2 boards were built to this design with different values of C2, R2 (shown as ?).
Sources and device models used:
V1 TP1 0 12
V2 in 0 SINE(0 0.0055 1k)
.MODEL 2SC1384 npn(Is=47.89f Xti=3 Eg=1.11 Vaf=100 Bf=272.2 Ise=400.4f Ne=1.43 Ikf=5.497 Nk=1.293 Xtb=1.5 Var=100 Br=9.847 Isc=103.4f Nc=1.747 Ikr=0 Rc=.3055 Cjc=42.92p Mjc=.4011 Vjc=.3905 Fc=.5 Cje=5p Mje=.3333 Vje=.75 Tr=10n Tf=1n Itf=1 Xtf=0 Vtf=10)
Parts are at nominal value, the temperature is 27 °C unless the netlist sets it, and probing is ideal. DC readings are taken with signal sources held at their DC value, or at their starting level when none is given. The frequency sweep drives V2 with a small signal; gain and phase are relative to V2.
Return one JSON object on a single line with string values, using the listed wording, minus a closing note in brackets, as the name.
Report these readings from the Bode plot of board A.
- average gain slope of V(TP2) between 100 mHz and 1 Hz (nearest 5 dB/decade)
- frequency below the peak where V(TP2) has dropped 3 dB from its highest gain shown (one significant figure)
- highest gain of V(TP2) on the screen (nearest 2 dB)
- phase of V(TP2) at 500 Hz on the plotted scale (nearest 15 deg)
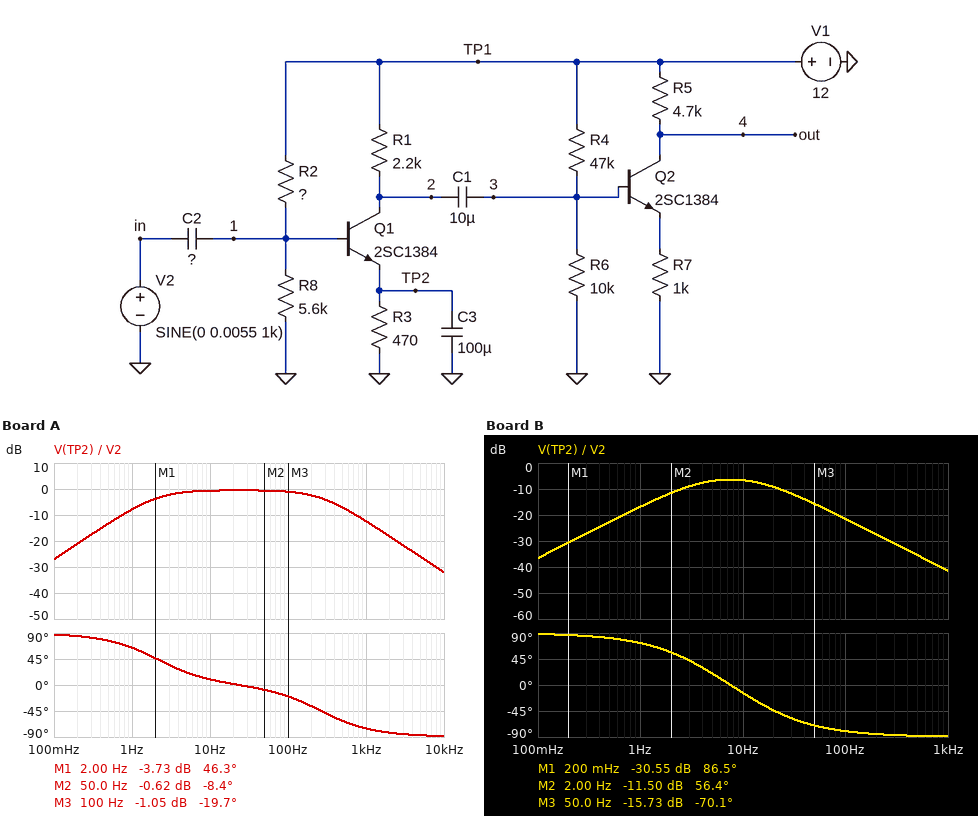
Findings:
{"average gain slope of V(TP2) between 100 mHz and 1 Hz": "20 dB/decade", "frequency below the peak where V(TP2) has dropped 3 dB from its highest gain shown": "2 Hz", "highest gain of V(TP2) on the screen": "0 dB", "phase of V(TP2) at 500 Hz on the plotted scale": "-60 deg"}
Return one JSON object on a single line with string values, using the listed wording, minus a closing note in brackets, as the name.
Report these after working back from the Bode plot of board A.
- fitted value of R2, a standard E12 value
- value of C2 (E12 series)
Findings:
{"fitted value of R2, a standard E12 value": "18 kΩ", "value of C2": "18 µF"}
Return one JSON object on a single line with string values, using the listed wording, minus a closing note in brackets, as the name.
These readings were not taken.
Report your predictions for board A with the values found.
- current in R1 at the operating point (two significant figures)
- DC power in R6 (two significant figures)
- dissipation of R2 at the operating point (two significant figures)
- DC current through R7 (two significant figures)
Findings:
{"current in R1 at the operating point": "4.3 mA", "DC power in R6": "400 µW", "dissipation of R2 at the operating point": "4.8 mW", "DC current through R7": "1.4 mA"}
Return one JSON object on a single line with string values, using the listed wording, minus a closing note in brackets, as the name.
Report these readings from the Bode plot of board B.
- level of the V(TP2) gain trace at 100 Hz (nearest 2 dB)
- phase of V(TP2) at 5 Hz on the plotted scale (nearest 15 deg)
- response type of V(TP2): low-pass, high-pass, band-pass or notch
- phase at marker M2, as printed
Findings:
{"level of the V(TP2) gain trace at 100 Hz": "-22 dB", "phase of V(TP2) at 5 Hz on the plotted scale": "15 deg", "response type of V(TP2): low-pass, high-pass, band-pass or notch": "band-pass", "phase at marker M2, as printed": "56.4 deg"}
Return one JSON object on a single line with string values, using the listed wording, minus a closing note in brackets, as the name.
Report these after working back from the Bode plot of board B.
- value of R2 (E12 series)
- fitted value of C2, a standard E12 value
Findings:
{"value of R2": "100 kΩ", "fitted value of C2, a standard E12 value": "6.8 µF"}
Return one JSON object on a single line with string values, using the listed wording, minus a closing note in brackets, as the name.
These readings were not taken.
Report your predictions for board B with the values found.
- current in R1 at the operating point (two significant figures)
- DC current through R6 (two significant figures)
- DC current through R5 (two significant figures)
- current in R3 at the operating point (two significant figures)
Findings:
{"current in R1 at the operating point": "140 µA", "DC current through R6": "200 µA", "DC current through R5": "1.4 mA", "current in R3 at the operating point": "140 µA"}
